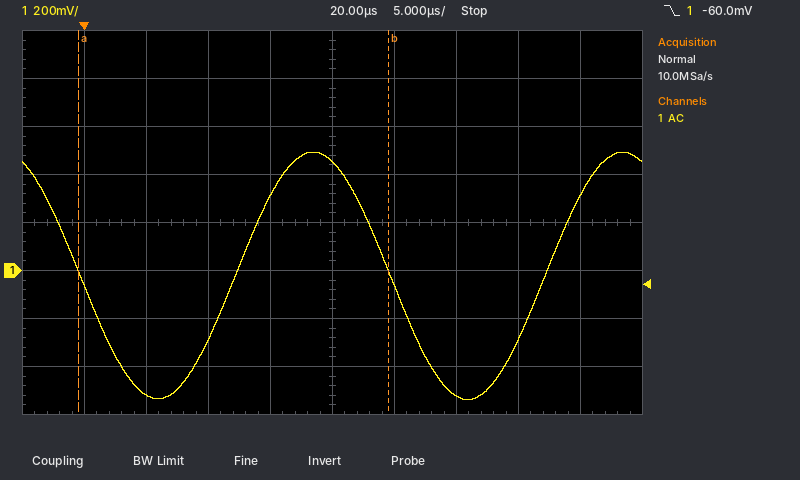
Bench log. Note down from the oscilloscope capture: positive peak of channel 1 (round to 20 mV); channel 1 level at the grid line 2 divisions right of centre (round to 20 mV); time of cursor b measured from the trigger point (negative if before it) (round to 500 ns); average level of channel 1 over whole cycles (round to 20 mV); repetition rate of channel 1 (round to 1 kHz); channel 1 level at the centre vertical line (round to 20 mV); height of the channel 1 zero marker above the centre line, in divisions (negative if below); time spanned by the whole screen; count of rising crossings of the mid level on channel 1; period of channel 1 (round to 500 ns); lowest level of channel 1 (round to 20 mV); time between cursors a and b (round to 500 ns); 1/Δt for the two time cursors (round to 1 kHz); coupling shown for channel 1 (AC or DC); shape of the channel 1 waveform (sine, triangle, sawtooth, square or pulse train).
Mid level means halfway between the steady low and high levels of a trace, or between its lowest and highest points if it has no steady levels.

500 mV
-520 mV
+24.5 µs
-20 mV
40 kHz
460 mV
-1.0 div
50 µs
2
25.0 µs
-540 mV
25.0 µs
40 kHz
AC
sine
